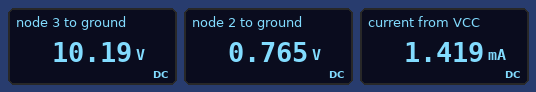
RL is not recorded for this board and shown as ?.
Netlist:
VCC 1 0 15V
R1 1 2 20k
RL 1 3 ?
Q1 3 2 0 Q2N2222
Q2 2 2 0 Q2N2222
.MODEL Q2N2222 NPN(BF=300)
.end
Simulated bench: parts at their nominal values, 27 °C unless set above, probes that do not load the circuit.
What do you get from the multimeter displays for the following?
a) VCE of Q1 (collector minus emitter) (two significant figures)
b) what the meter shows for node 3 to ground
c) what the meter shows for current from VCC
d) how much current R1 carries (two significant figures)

10 V
10.19 V
1.419 mA
710 µA
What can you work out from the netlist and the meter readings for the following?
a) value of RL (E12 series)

6.8 kΩ
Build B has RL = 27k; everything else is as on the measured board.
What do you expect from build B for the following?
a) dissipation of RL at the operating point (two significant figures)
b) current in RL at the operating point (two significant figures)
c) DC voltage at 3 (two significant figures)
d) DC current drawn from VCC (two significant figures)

8.3 mW
550 µA
66 mV
1.3 mA
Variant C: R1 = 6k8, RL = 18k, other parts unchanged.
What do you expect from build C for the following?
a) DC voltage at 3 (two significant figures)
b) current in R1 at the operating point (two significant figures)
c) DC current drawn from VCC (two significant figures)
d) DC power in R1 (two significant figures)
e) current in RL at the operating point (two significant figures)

36 mV
2.1 mA
2.9 mA
30 mW
830 µA
